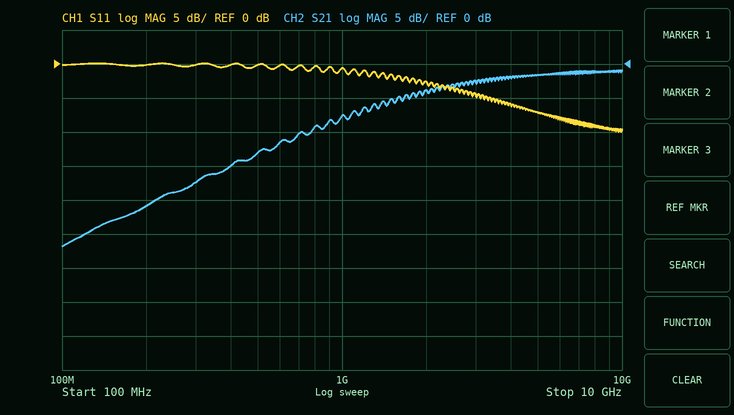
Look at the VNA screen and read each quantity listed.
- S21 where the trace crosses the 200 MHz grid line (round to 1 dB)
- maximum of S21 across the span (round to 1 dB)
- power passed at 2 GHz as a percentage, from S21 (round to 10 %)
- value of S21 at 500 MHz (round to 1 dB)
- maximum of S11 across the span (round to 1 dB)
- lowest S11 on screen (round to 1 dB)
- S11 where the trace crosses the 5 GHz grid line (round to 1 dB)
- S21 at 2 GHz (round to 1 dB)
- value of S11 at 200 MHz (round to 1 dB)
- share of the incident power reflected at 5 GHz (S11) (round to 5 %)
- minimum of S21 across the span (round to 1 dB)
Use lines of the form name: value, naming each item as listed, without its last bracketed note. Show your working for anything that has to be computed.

S21 where the trace crosses the 200 MHz grid line: -21 dB
maximum of S21 across the span: -1 dB
power passed at 2 GHz as a percentage, from S21: 10^(-4/10) ≈ 40 %
value of S21 at 500 MHz: -13 dB
maximum of S11 across the span: 0 dB
lowest S11 on screen: -10 dB
S11 where the trace crosses the 5 GHz grid line: -7 dB
S21 at 2 GHz: -4 dB
value of S11 at 200 MHz: 0 dB
share of the incident power reflected at 5 GHz (S11): 10^(-7/10) ≈ 20 %
minimum of S21 across the span: -27 dB
